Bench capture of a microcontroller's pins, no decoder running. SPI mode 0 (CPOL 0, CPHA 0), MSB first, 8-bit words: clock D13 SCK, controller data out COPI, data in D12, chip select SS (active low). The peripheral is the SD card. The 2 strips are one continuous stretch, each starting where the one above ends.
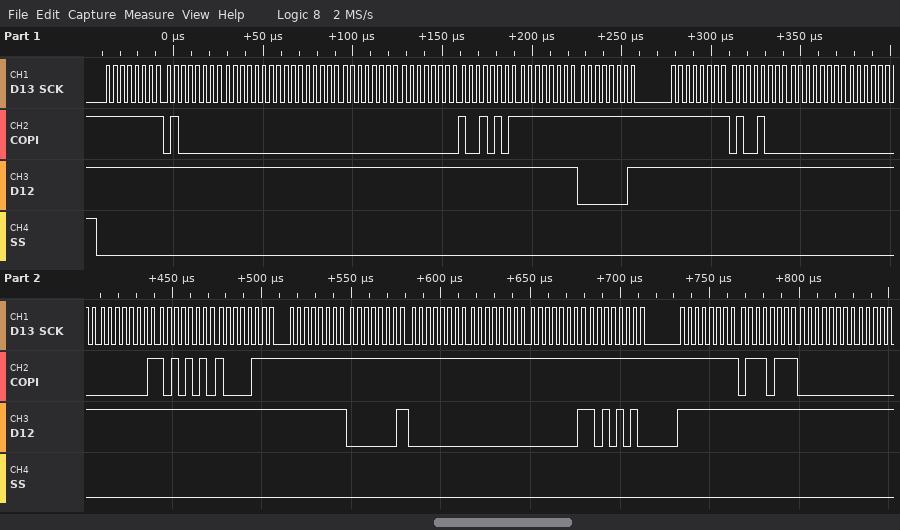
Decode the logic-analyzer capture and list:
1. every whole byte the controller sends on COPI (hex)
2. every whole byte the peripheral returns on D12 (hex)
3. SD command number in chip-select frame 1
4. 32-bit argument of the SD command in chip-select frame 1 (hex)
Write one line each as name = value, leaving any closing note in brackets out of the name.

every whole byte the controller sends on COPI = FF 40 00 00 00 00 95 FF FF FF 48 00 00 01 AA 87 FF FF FF FF FF FF FF 77 00
every whole byte the peripheral returns on D12 = FF FF FF FF FF FF FF FF 01 FF FF FF FF FF FF FF FF 01 00 00 01 AA FF FF FF
SD command number in chip-select frame 1 = CMD0
32-bit argument of the SD command in chip-select frame 1 = 0x00000000
